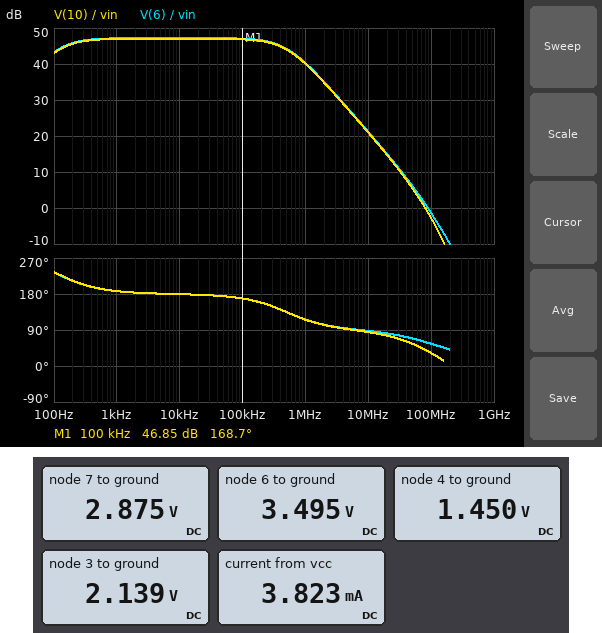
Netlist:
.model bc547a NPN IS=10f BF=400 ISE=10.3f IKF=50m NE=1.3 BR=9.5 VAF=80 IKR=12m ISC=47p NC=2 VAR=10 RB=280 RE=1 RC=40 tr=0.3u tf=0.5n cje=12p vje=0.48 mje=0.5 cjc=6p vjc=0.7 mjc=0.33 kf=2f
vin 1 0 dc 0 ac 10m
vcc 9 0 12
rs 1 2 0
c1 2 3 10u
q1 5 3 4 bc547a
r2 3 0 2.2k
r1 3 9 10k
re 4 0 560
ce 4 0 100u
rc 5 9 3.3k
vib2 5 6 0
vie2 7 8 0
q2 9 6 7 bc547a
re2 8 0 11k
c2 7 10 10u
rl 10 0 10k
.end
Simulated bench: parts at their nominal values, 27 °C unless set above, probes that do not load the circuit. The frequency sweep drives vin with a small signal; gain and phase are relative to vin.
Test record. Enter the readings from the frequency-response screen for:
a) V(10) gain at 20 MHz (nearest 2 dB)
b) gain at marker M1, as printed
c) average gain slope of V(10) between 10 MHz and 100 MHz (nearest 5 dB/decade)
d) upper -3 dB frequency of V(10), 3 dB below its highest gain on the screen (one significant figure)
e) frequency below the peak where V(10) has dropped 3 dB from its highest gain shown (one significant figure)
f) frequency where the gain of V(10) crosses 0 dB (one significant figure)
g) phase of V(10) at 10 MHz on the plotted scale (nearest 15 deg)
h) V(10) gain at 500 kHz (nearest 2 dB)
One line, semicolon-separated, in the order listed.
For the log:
14 dB; 46.85 dB; -25 dB/decade; 500 kHz; 100 Hz; 80 MHz; 90 deg; 44 dB
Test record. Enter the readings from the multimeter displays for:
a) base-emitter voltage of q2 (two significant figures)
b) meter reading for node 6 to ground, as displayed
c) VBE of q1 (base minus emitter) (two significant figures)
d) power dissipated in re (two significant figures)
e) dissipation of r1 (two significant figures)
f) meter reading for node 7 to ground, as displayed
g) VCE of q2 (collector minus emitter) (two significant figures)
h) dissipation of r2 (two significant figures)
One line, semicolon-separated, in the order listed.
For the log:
620 mV; 3.495 V; 690 mV; 3.8 mW; 9.7 mW; 2.875 V; 9.1 V; 2.1 mW
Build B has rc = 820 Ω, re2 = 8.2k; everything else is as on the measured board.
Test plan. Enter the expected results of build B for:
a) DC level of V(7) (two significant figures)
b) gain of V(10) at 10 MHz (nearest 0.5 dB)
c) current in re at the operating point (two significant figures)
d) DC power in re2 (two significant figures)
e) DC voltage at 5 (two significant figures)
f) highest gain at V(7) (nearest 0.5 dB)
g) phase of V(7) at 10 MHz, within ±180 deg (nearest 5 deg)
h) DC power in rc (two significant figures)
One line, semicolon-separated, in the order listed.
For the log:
9.2 V; 22.5 dB; 2.6 mA; 10 mW; 9.9 V; 36.0 dB; 95 deg; 5.5 mW
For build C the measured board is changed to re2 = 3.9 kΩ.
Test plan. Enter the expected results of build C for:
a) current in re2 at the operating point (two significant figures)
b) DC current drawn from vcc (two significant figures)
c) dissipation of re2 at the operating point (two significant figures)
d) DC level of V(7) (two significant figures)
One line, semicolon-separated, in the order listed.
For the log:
730 µA; 4.3 mA; 2.1 mW; 2.8 V
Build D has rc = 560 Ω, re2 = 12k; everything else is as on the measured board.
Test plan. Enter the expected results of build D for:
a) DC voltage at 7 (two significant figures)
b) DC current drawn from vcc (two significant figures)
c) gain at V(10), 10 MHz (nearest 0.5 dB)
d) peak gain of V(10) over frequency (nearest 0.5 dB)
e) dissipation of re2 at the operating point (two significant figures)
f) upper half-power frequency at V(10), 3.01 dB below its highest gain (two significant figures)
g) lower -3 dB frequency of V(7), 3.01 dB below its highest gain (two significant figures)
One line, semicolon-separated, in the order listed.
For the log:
9.9 V; 4.4 mA; 21.5 dB; 32.5 dB; 8.2 mW; 2.9 MHz; 130 Hz
